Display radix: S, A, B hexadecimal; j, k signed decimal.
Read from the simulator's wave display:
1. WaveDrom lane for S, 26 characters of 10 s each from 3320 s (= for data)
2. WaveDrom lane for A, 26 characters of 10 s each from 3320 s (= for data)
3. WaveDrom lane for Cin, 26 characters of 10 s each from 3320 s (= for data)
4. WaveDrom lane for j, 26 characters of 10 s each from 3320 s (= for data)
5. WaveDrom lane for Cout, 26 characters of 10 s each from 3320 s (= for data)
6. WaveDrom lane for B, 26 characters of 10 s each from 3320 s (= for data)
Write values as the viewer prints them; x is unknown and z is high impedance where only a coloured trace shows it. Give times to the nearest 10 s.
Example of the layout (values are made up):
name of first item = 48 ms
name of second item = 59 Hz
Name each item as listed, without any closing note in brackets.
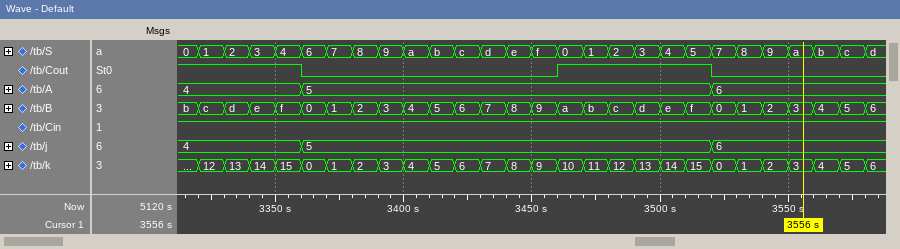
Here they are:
WaveDrom lane for S, 26 characters of 10 s each from 3320 s = {name: 'S', wave: '==========================', data: '1 2 3 4 6 7 8 9 a b c d e f 0 1 2 3 4 5 7 8 9 a b c'}
WaveDrom lane for A, 26 characters of 10 s each from 3320 s = {name: 'A', wave: '=...=...............=.....', data: '4 5 6'}
WaveDrom lane for Cin, 26 characters of 10 s each from 3320 s = {name: 'Cin', wave: '1.........................'}
WaveDrom lane for j, 26 characters of 10 s each from 3320 s = {name: 'j', wave: '=...=...............=.....', data: '4 5 6'}
WaveDrom lane for Cout, 26 characters of 10 s each from 3320 s = {name: 'Cout', wave: '1...0.........1.....0.....'}
WaveDrom lane for B, 26 characters of 10 s each from 3320 s = {name: 'B', wave: '==========================', data: 'c d e f 0 1 2 3 4 5 6 7 8 9 a b c d e f 0 1 2 3 4 5'}
